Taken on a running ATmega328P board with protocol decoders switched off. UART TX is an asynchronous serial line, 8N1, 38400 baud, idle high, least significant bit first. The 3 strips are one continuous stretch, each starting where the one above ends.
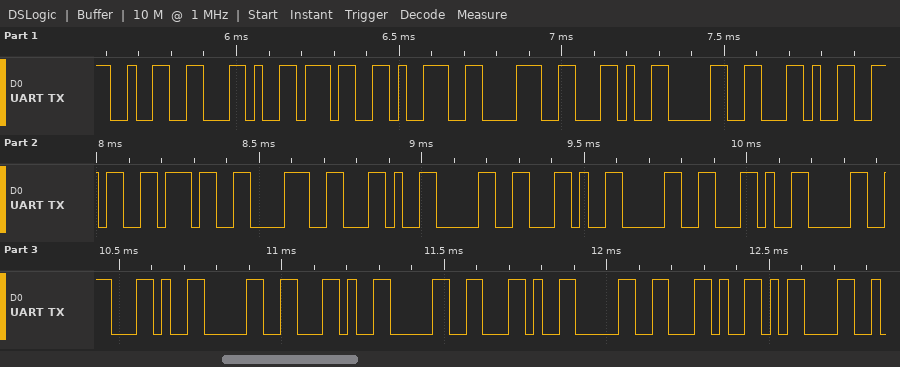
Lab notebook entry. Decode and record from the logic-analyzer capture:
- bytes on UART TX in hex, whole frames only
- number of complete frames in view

32 2C 37 39 38 2C 30 2C 36 37 38 2C 30 2C 30 2C 30 2C 30 2C 30 2C 30 2C 0D
25
